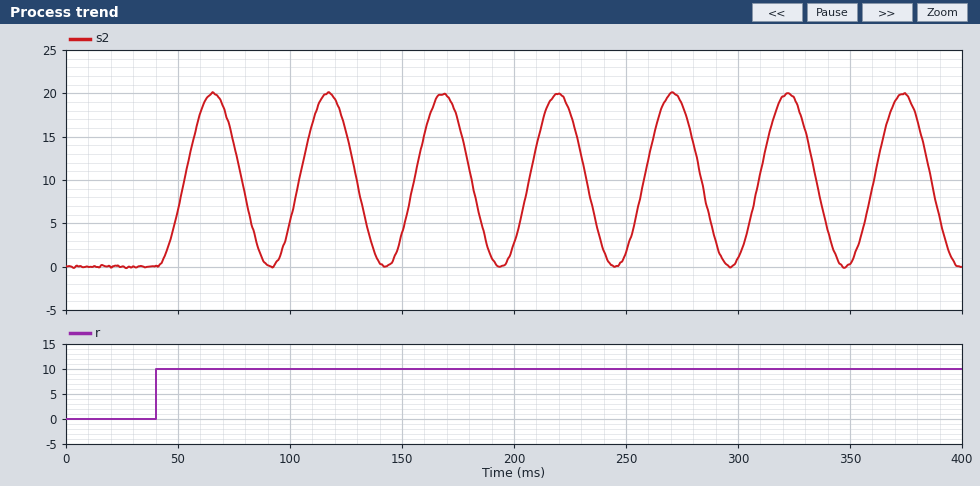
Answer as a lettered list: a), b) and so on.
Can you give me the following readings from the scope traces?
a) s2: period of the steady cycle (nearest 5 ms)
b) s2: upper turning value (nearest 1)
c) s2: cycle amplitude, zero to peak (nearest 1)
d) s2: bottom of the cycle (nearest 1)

a) 50 ms
b) 20
c) 10
d) 0
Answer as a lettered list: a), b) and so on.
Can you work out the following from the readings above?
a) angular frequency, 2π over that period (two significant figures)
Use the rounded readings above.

a) 0.13 rad/ms
